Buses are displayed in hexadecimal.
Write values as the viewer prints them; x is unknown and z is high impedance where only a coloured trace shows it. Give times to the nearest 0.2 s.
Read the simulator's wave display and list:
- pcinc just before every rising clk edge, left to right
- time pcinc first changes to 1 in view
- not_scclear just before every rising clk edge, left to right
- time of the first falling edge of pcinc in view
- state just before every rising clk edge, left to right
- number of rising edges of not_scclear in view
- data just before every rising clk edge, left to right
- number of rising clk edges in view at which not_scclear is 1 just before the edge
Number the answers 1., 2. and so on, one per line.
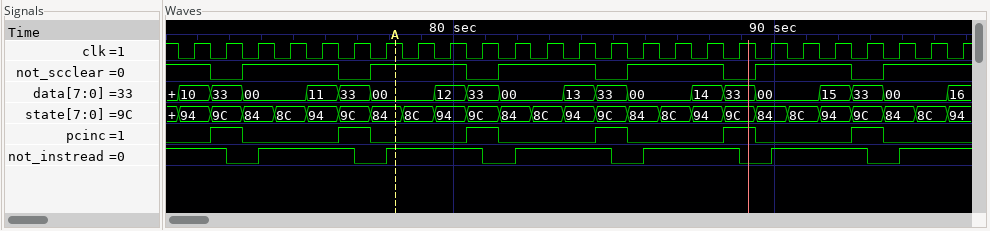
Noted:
1. 0 1 0 0 0 1 0 0 0 1 0 0 0 1 0 0 0 1 0 0 0 1 0 0 0
2. 72.4 s
3. 1 0 1 1 1 0 1 1 1 0 1 1 1 0 1 1 1 0 1 1 1 0 1 1 1
4. 73.4 s
5. 94, 9C, 84, 8C, 94, 9C, 84, 8C, 94, 9C, 84, 8C, 94, 9C, 84, 8C, 94, 9C, 84, 8C, 94, 9C, 84, 8C, 94
6. 6
7. 10, 33, 00, 00, 11, 33, 00, 00, 12, 33, 00, 00, 13, 33, 00, 00, 14, 33, 00, 00, 15, 33, 00, 00, 16
8. 19
